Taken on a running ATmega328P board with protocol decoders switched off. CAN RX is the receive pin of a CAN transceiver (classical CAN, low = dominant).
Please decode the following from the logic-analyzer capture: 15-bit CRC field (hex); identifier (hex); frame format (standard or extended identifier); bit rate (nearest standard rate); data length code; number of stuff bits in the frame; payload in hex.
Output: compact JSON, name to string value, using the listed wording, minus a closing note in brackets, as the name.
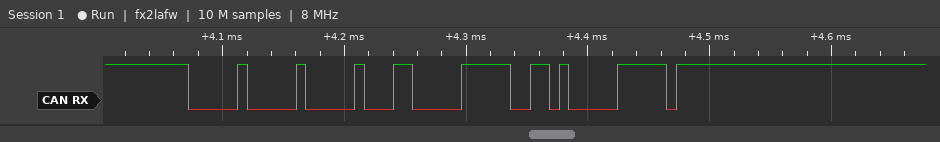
{"15-bit CRC field": "0x6D07", "identifier": "0x000", "frame format": "standard", "bit rate": "125 kbit/s", "data length code": "1", "number of stuff bits in the frame": "6", "payload in hex": "83"}
